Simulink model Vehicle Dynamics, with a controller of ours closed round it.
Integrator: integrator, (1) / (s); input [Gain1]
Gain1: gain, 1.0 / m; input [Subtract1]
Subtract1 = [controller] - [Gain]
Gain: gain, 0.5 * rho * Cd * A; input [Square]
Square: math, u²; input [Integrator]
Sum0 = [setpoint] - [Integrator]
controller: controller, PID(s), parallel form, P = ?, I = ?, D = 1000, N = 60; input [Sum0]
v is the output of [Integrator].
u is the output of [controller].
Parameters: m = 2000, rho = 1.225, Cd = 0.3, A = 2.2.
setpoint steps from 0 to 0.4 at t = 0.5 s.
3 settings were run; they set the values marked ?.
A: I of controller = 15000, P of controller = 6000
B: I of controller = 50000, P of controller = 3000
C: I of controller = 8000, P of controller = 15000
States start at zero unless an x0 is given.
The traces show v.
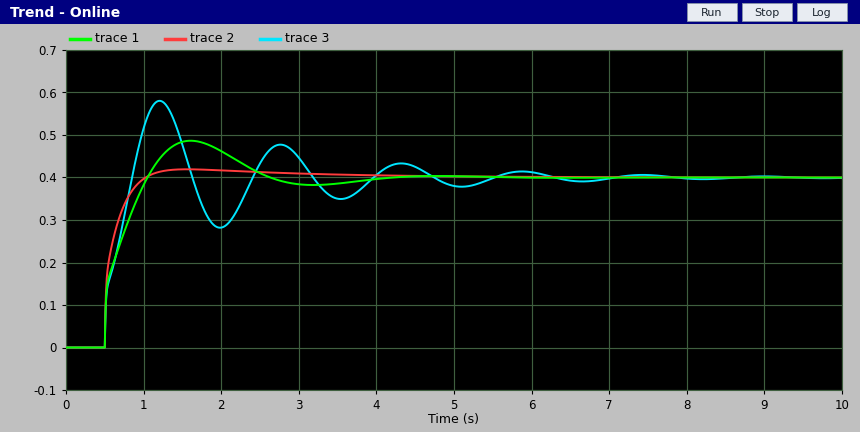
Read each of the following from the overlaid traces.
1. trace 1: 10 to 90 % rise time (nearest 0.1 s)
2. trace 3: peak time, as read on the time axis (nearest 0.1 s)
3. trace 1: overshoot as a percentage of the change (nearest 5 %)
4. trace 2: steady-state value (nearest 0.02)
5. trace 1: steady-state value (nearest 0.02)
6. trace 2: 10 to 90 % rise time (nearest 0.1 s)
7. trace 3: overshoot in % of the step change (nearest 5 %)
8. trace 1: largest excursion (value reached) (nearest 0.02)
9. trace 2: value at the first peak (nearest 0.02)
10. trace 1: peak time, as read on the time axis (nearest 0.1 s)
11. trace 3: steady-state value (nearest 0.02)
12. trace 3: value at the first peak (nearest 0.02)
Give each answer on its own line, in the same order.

0.4 s
1.2 s
20 %
0.40
0.40
0.3 s
45 %
0.48
0.42
1.6 s
0.40
0.58
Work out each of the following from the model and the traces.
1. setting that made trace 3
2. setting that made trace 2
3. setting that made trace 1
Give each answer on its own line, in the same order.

B
C
A
